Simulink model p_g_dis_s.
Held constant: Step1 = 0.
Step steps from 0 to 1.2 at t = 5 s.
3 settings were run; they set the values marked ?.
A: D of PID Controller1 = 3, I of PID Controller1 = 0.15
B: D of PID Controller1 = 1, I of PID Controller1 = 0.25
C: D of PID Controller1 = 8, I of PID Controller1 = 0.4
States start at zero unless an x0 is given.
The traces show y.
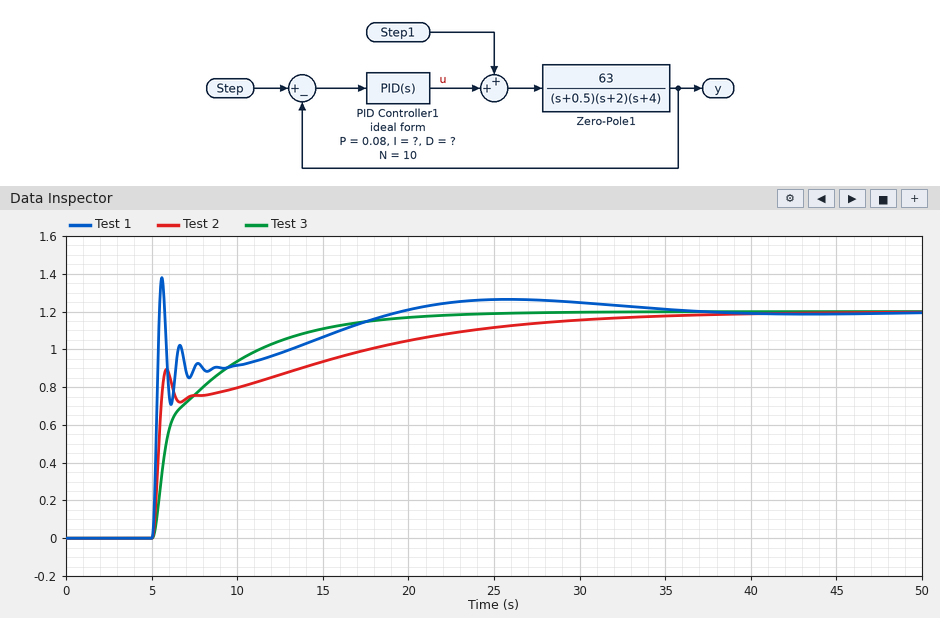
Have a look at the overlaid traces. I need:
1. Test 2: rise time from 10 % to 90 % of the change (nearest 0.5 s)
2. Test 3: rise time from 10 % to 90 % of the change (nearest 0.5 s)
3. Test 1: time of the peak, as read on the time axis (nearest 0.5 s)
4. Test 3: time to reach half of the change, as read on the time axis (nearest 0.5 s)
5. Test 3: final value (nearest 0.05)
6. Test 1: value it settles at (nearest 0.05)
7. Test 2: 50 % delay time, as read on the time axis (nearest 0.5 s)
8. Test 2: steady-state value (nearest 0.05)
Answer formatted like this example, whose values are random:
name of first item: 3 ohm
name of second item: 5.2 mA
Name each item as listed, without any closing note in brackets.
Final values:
Test 2: rise time from 10 % to 90 % of the change: 17.0 s
Test 3: rise time from 10 % to 90 % of the change: 8.5 s
Test 1: time of the peak, as read on the time axis: 5.5 s
Test 3: time to reach half of the change, as read on the time axis: 6.0 s
Test 3: final value: 1.20
Test 1: value it settles at: 1.20
Test 2: 50 % delay time, as read on the time axis: 5.5 s
Test 2: steady-state value: 1.20
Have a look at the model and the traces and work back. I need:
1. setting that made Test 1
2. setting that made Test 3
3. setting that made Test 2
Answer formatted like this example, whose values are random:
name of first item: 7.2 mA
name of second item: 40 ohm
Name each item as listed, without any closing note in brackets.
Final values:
setting that made Test 1: C
setting that made Test 3: B
setting that made Test 2: A
